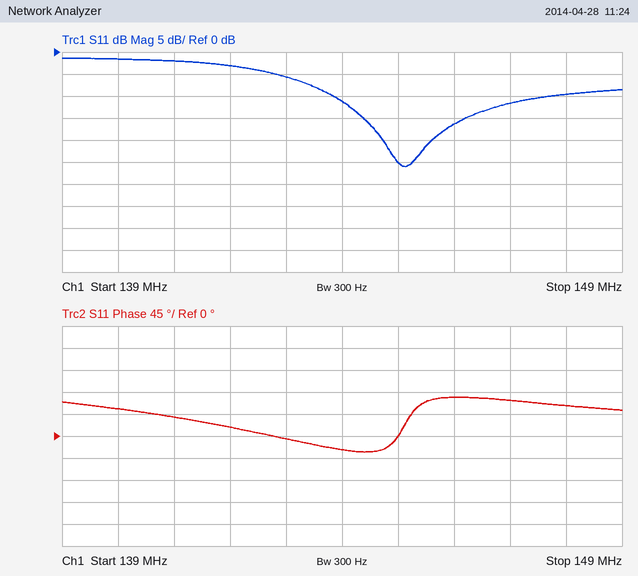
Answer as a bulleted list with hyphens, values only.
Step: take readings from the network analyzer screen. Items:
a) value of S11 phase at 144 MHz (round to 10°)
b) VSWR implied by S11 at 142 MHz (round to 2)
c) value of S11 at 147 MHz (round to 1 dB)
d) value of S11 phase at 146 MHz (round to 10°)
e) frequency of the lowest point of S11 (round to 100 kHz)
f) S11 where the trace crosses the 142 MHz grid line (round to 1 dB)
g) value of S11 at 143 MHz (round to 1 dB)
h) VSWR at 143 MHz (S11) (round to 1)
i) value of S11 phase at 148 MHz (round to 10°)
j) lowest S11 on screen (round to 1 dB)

- -30°
- 6
- -12 dB
- 80°
- 145.1 MHz
- -3 dB
- -6 dB
- 3
- 60°
- -26 dB
